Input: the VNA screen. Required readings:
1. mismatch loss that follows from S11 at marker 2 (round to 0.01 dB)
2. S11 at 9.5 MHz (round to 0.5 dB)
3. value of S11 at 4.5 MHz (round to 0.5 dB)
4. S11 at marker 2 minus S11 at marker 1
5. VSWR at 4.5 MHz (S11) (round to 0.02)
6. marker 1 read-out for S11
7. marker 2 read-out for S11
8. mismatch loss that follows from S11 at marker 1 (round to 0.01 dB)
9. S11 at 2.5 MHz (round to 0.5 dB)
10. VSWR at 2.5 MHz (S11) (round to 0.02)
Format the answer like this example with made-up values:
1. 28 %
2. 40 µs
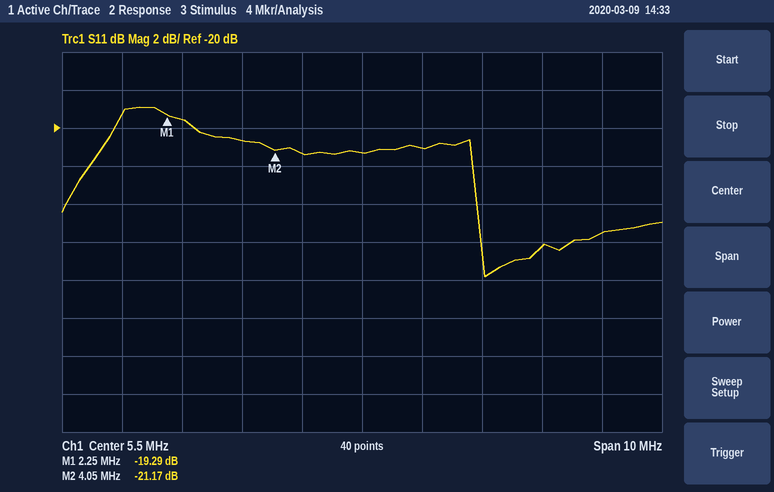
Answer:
1. 0.03 dB
2. -25.5 dB
3. -21.5 dB
4. -1.88 dB
5. 1.18
6. -19.29 dB
7. -21.17 dB
8. 0.05 dB
9. -19.5 dB
10. 1.24
